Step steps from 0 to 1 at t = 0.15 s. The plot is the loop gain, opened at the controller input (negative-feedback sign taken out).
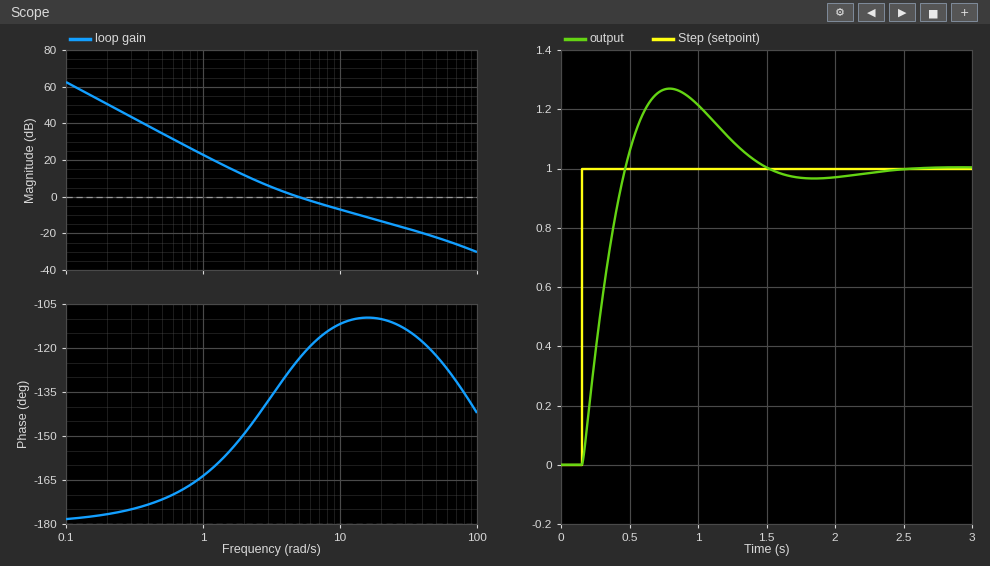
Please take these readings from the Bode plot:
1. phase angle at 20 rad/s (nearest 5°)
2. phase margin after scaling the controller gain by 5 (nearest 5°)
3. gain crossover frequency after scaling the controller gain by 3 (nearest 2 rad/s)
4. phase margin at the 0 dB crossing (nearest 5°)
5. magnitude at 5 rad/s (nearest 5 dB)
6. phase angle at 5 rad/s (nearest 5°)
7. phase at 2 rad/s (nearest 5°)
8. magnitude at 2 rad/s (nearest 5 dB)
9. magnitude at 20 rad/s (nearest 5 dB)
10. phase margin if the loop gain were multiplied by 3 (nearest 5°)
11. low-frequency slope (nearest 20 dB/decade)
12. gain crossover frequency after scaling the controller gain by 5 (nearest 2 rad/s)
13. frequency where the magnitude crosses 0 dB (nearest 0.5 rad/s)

-110°
70°
14 rad/s
55°
0 dB
-125°
-150°
10 dB
-15 dB
70°
-40 dB/decade
22 rad/s
5.0 rad/s
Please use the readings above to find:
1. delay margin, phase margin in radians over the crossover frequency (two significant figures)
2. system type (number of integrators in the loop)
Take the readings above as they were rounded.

0.19 s
2
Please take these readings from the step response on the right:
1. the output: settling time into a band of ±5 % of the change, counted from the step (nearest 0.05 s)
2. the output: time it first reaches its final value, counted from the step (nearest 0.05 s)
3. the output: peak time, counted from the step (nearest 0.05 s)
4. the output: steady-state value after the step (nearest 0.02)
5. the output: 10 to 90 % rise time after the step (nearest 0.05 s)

1.20 s
0.30 s
0.65 s
1.00
0.25 s
